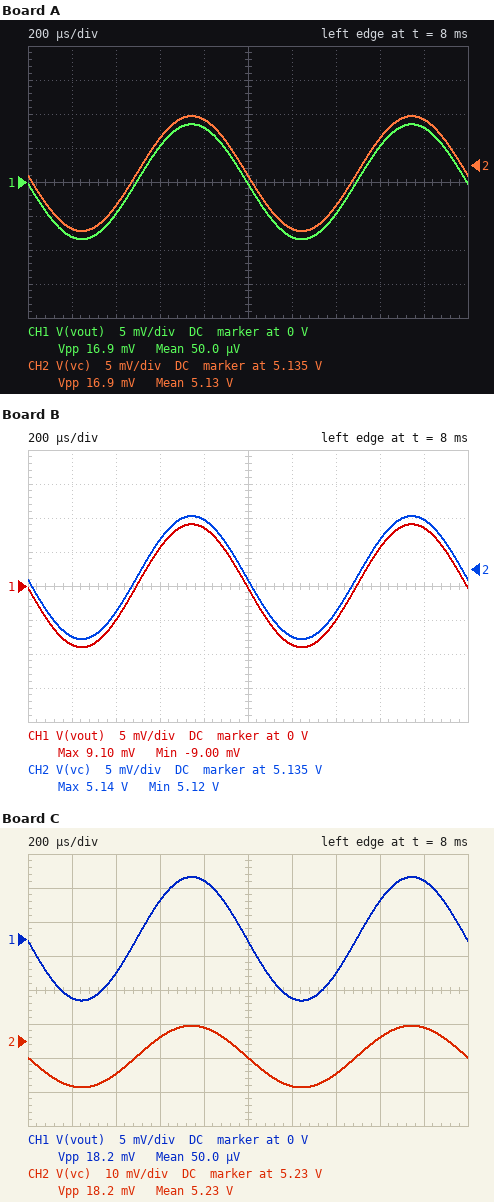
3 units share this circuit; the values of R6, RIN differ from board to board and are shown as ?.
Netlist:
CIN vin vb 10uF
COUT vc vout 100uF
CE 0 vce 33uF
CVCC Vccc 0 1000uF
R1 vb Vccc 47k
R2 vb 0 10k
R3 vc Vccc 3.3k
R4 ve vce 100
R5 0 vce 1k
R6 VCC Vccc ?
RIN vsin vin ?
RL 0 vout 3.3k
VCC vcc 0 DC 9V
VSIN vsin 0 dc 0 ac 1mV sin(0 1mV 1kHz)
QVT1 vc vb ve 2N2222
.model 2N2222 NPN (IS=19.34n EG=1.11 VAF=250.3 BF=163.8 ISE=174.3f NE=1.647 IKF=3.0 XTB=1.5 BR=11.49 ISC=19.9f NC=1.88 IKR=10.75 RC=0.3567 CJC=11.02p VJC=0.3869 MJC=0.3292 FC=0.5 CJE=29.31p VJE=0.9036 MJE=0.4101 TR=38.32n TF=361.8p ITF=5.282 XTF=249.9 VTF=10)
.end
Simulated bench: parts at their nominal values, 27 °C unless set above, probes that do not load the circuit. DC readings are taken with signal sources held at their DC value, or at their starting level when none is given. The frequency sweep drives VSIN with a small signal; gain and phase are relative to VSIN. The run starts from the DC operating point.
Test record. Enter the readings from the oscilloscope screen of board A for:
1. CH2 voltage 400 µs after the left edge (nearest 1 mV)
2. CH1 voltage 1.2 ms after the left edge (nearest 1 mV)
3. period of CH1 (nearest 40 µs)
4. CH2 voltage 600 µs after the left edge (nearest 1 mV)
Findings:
5.129 V
-8 mV
1.00 ms
5.139 V
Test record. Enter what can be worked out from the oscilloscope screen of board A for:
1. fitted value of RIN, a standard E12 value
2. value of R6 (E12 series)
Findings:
3.3 kΩ
270 Ω
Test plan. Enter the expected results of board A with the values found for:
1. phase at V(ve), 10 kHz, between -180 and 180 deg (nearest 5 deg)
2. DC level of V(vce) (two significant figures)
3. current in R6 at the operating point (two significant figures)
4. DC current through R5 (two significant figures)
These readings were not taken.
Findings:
0 deg
1.1 V
1.2 mA
1.1 mA
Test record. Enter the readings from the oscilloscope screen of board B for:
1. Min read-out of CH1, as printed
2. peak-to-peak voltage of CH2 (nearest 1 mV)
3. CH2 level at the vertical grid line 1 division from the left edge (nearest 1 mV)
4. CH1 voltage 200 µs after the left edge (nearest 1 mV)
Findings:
-9.00 mV
18 mV
5.125 V
-9 mV
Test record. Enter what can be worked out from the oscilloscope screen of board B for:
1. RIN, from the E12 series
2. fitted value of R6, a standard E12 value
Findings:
2.7 kΩ
270 Ω
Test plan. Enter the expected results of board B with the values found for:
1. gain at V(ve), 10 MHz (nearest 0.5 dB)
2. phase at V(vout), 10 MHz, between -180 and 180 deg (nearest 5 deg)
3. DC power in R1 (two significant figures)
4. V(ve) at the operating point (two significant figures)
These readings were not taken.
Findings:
-24.0 dB
90 deg
1.1 mW
1.2 V
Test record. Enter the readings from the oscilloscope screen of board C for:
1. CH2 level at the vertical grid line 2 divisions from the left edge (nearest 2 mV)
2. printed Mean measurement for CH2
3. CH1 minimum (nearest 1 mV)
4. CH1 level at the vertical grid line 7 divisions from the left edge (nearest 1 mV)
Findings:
5.220 V
5.23 V
-9 mV
-5 mV
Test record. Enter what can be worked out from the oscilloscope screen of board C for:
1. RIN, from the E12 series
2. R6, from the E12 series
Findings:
2.7 kΩ
120 Ω
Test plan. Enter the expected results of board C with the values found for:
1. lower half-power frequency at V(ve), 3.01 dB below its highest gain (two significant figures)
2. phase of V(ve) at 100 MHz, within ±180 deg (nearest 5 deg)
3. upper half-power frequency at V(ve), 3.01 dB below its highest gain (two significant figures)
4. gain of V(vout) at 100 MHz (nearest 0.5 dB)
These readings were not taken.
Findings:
1.4 Hz
-5 deg
480 kHz
-20.0 dB
